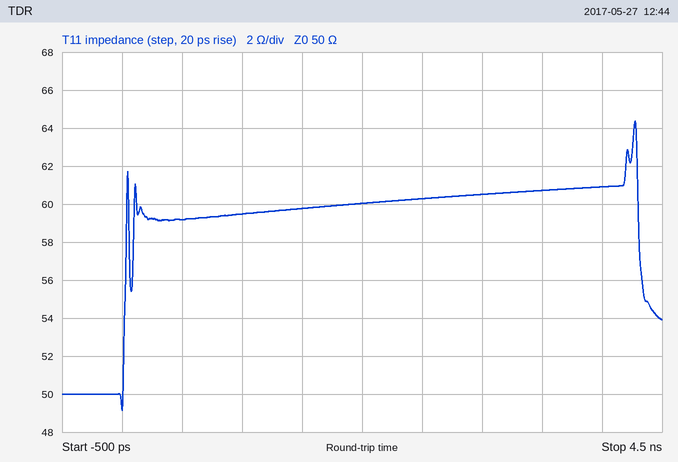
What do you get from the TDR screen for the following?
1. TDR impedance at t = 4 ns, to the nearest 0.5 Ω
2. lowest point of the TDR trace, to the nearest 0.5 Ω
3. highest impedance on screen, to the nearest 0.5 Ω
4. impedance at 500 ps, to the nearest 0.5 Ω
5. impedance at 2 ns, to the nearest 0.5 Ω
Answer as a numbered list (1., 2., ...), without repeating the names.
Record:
1. 61.0 Ω
2. 49.0 Ω
3. 64.5 Ω
4. 59.0 Ω
5. 60.0 Ω
